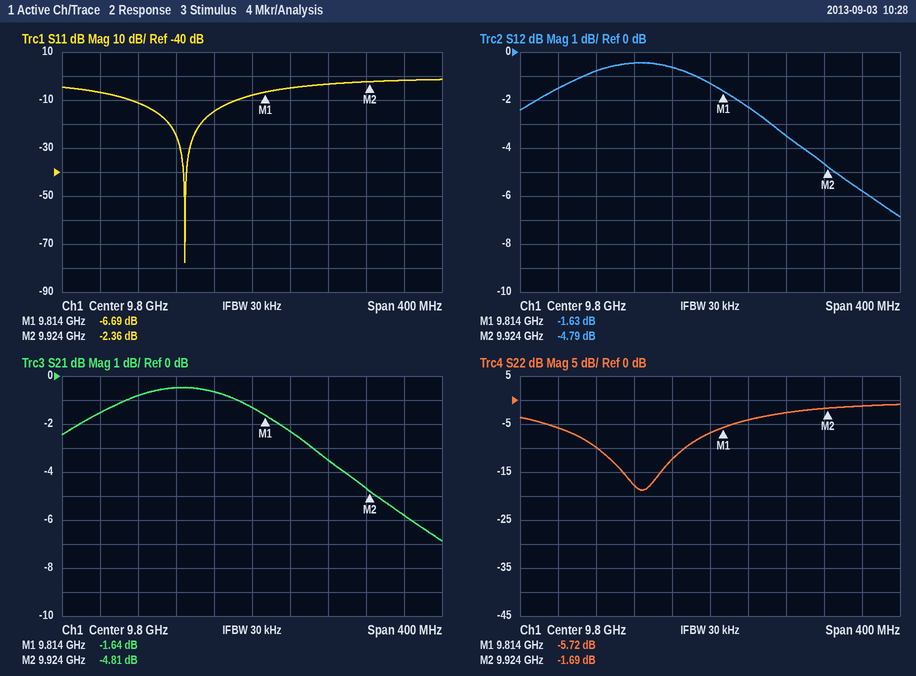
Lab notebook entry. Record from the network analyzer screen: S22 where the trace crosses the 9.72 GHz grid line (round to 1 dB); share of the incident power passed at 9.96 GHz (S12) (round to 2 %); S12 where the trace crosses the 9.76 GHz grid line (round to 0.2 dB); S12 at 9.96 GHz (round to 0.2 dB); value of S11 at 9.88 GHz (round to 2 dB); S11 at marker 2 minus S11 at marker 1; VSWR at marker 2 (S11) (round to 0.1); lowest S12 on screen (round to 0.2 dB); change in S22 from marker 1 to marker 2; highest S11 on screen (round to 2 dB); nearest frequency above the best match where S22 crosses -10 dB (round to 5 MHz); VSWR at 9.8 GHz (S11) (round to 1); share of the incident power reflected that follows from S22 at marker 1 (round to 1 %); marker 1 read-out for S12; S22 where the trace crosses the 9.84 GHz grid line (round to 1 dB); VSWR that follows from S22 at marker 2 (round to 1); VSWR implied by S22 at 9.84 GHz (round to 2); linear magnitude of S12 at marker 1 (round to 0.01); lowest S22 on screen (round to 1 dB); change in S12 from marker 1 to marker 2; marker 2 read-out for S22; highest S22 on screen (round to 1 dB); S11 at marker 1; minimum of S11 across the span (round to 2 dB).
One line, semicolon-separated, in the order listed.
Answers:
-18 dB; 26 %; -0.6 dB; -5.8 dB; -4 dB; 4.33 dB; 7.4; -6.8 dB; 4.03 dB; -2 dB; 9.775 GHz; 2; 27 %; -1.63 dB; -4 dB; 10; 4; 0.83; -19 dB; -3.16 dB; -1.69 dB; -1 dB; -6.69 dB; -78 dB
